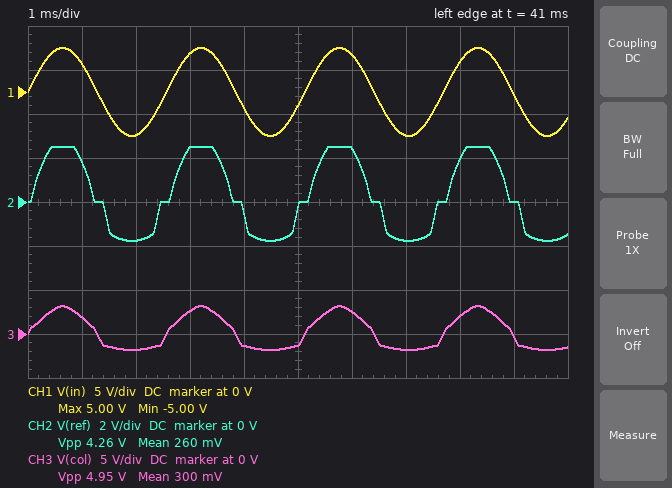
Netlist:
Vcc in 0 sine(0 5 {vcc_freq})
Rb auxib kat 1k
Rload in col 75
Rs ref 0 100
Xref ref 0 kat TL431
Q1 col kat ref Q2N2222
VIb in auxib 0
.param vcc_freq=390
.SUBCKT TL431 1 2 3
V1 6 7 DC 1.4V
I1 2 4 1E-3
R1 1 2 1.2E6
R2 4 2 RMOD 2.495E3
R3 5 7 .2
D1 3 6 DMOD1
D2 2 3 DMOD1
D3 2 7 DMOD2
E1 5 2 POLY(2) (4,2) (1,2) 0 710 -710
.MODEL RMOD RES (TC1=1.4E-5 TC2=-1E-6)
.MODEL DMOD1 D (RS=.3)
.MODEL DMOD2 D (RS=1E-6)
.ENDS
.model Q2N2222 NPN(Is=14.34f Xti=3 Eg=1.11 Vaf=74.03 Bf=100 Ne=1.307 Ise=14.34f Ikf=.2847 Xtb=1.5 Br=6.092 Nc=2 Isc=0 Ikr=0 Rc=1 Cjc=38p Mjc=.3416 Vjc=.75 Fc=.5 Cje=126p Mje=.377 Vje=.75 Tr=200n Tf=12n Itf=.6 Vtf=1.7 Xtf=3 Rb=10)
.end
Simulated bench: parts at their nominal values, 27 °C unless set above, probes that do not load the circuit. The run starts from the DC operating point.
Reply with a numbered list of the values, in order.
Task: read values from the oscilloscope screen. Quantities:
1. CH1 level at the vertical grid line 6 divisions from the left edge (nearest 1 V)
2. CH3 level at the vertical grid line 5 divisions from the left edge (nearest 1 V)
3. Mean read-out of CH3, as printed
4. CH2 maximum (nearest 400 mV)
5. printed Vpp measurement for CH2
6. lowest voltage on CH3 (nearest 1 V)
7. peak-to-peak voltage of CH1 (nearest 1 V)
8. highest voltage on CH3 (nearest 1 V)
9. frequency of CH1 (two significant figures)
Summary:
1. 4 V
2. -1 V
3. 300 mV
4. 2.4 V
5. 4.26 V
6. -2 V
7. 10 V
8. 3 V
9. 390 Hz
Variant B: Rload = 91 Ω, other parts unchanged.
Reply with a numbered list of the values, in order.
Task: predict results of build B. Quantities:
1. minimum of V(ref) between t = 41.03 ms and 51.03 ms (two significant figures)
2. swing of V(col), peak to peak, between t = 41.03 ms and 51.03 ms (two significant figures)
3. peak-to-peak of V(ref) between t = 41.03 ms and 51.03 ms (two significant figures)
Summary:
1. -1.7 V
2. 4.5 V
3. 4.2 V
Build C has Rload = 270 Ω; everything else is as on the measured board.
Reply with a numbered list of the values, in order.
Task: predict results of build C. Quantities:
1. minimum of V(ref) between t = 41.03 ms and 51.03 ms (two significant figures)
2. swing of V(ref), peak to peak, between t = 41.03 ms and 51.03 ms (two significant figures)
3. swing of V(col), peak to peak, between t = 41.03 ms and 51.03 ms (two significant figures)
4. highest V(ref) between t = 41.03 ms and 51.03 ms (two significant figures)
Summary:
1. -1.1 V
2. 2.7 V
3. 3.0 V
4. 1.5 V
